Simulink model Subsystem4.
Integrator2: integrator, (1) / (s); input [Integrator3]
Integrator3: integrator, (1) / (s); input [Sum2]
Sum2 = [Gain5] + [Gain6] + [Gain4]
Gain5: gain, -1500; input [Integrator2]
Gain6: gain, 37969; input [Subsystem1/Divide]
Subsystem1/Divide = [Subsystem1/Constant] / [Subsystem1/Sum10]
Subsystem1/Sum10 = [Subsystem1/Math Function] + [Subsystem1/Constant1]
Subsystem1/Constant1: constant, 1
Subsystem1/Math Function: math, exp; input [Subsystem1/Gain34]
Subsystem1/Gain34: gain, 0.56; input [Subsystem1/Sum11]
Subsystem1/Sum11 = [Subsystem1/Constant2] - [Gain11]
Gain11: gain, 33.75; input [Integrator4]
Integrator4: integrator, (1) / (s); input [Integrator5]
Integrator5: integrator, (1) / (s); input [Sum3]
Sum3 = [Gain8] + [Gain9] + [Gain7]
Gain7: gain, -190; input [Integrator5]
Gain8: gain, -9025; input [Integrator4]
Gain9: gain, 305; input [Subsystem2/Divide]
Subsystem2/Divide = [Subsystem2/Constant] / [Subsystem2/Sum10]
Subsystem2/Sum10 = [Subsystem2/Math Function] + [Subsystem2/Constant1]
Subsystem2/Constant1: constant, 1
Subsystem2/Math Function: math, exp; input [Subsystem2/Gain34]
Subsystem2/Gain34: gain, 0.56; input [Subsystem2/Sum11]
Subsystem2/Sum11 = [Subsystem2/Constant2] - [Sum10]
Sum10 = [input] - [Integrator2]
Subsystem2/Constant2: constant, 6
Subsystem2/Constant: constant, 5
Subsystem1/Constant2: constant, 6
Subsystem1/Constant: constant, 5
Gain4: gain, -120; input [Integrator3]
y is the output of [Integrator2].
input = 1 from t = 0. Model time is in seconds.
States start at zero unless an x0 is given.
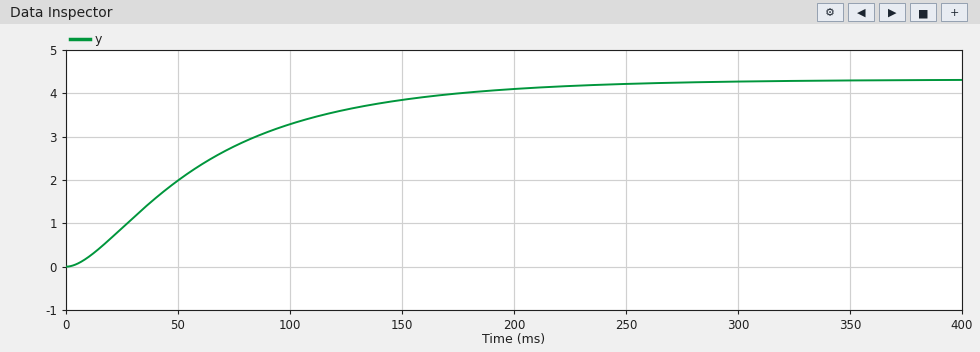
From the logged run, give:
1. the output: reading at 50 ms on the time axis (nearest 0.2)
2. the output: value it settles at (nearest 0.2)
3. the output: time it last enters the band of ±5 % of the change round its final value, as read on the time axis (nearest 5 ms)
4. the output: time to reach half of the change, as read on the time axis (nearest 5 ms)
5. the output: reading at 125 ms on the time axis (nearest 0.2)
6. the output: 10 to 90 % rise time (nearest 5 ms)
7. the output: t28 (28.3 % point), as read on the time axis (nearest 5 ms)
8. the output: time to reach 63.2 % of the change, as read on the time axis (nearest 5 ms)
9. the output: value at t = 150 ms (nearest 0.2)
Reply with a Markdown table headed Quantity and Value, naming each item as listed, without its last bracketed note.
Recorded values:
| Quantity | Value |
|---|---|
| the output: reading at 50 ms on the time axis | 2.0 |
| the output: value it settles at | 4.4 |
| the output: time it last enters the band of ±5 % of the change round its final value, as read on the time axis | 200 ms |
| the output: time to reach half of the change, as read on the time axis | 55 ms |
| the output: reading at 125 ms on the time axis | 3.6 |
| the output: 10 to 90 % rise time | 140 ms |
| the output: t28 (28.3 % point), as read on the time axis | 30 ms |
| the output: time to reach 63.2 % of the change, as read on the time axis | 75 ms |
| the output: value at t = 150 ms | 3.8 |
